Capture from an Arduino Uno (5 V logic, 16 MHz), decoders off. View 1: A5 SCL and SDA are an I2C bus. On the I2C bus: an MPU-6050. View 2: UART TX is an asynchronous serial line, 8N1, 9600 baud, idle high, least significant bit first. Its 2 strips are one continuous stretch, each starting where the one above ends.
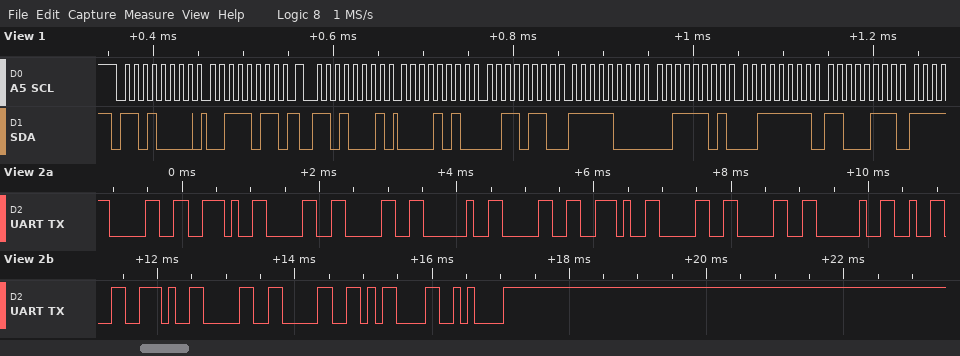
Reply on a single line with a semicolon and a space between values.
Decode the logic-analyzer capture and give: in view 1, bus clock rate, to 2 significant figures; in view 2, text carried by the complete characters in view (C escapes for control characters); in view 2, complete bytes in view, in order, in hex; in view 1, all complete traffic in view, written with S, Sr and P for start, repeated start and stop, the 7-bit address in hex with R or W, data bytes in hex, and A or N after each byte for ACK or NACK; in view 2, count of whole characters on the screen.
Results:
100 kHz; "0.00 0.00 2.00\r\n"; 30 2E 30 30 20 30 2E 30 30 20 32 2E 30 30 0D 0A; S 68W A 3B A Sr 68R A 0A A 36 A F8 A 3D A 3F A C7 A; 16
